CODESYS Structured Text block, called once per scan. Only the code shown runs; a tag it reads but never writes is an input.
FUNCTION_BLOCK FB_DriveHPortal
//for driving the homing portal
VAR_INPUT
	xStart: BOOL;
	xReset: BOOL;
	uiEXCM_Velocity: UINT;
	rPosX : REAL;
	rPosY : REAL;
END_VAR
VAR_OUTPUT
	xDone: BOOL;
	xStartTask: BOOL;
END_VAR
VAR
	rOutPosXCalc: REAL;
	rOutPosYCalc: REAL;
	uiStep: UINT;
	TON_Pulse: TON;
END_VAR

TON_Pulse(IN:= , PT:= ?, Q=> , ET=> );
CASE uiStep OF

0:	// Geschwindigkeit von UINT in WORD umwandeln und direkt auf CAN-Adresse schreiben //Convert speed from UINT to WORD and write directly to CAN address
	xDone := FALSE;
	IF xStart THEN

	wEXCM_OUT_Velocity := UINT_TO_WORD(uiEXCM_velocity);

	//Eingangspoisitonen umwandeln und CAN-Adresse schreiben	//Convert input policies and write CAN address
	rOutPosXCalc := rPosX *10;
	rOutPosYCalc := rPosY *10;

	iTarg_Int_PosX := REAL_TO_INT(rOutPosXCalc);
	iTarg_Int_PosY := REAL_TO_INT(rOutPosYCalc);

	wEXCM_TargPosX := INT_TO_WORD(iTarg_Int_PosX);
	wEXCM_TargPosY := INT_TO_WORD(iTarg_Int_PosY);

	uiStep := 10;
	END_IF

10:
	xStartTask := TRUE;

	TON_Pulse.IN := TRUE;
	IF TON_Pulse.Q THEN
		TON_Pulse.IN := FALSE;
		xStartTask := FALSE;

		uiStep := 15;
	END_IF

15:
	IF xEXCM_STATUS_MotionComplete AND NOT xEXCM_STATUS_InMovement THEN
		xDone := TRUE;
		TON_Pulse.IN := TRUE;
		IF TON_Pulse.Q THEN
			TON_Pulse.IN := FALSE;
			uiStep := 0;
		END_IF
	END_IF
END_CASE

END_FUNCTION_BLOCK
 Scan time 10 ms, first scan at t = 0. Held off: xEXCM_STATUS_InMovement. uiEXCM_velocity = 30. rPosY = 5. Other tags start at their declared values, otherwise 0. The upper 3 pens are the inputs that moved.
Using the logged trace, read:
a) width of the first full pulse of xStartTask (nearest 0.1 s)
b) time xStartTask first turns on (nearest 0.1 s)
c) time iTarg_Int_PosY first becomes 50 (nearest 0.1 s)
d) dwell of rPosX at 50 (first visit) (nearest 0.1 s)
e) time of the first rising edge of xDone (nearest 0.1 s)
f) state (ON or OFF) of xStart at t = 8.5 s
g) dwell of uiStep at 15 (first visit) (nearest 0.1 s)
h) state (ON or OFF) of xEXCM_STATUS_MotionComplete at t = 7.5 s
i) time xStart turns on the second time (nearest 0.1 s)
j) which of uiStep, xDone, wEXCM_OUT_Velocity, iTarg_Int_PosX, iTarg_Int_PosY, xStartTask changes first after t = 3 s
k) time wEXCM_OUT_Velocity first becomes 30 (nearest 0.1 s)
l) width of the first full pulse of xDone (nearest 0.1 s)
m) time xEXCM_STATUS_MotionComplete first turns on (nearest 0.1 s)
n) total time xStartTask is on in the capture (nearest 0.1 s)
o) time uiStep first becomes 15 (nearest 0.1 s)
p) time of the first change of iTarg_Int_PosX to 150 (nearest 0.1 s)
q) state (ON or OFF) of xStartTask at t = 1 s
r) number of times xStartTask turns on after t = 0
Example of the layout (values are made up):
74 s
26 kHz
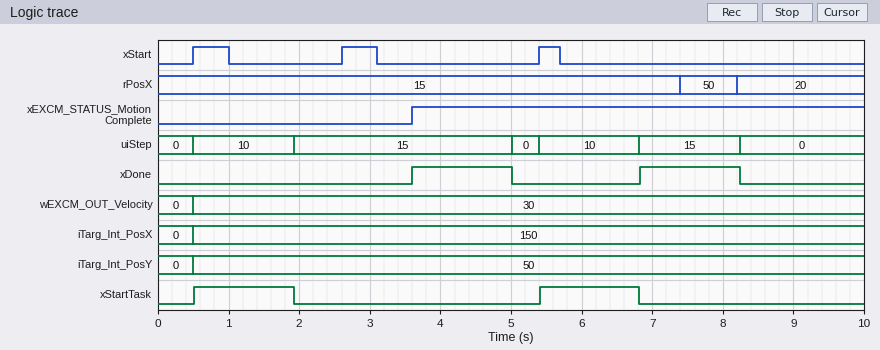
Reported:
1.4 s
0.5 s
0.5 s
0.8 s
3.6 s
OFF
3.1 s
ON
2.6 s
xDone
0.5 s
1.4 s
3.6 s
2.8 s
1.9 s
0.5 s
ON
2
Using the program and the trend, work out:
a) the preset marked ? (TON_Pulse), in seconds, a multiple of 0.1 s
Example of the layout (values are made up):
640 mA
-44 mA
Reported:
1.4 s
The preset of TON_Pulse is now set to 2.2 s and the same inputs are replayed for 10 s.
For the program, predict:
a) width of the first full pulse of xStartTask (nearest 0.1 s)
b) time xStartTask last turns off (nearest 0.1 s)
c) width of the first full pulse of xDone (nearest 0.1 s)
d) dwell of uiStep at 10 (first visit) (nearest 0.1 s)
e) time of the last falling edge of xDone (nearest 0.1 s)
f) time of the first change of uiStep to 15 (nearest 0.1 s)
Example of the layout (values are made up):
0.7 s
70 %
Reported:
2.2 s
2.7 s
2.2 s
2.2 s
5.8 s
2.7 s
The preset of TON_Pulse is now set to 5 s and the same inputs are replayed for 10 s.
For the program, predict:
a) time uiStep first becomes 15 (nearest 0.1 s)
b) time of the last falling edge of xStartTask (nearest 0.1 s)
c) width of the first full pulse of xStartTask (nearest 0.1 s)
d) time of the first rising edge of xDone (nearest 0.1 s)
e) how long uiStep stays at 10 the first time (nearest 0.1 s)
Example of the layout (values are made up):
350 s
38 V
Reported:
5.5 s
5.5 s
5.0 s
5.5 s
5.0 s
